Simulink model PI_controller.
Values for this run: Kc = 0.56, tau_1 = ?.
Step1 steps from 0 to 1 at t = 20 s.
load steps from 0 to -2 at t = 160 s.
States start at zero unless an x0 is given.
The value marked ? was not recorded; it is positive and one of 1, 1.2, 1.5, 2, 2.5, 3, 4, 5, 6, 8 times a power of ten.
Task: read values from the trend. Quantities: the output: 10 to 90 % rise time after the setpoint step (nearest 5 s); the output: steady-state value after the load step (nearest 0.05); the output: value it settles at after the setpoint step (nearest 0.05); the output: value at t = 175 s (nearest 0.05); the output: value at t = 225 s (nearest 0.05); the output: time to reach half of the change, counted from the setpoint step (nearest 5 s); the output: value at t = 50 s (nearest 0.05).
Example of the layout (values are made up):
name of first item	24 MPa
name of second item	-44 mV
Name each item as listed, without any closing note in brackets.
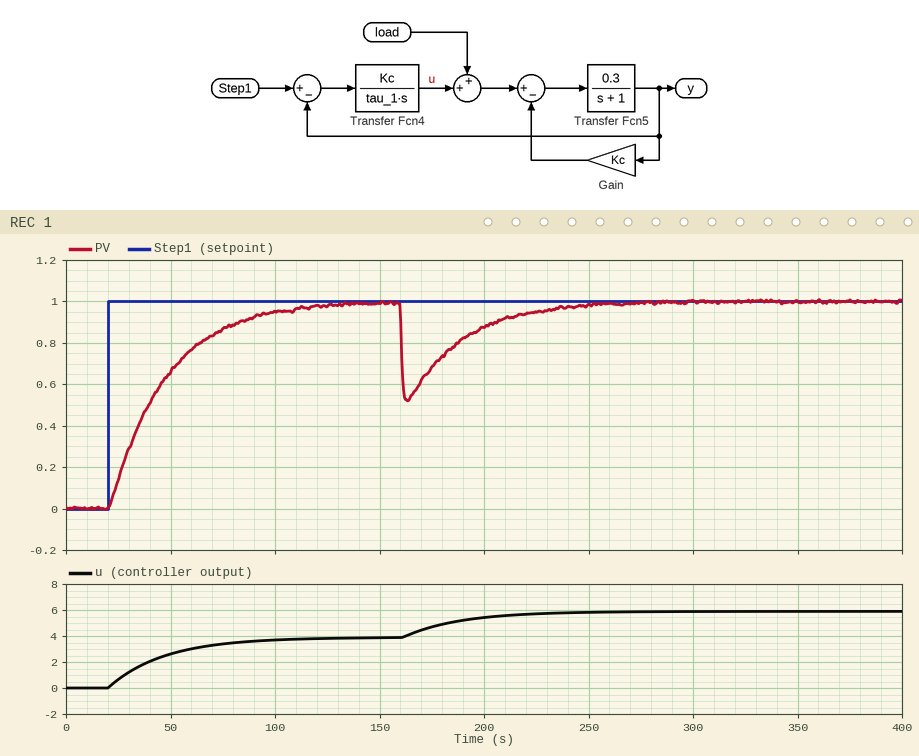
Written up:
the output: 10 to 90 % rise time after the setpoint step	60 s
the output: steady-state value after the load step	1.00
the output: value it settles at after the setpoint step	1.00
the output: value at t = 175 s	0.70
the output: value at t = 225 s	0.95
the output: time to reach half of the change, counted from the setpoint step	20 s
the output: value at t = 50 s	0.65
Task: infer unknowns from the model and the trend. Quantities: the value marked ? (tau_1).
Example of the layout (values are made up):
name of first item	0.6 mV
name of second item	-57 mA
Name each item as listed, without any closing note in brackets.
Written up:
the value marked ?	4
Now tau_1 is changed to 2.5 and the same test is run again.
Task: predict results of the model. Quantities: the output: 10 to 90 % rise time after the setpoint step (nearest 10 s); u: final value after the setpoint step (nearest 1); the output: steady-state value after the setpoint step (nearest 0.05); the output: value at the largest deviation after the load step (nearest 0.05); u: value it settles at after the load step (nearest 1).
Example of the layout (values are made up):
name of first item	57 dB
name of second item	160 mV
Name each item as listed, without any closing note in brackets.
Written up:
the output: 10 to 90 % rise time after the setpoint step	40 s
u: final value after the setpoint step	4
the output: steady-state value after the setpoint step	1.00
the output: value at the largest deviation after the load step	0.55
u: value it settles at after the load step	6
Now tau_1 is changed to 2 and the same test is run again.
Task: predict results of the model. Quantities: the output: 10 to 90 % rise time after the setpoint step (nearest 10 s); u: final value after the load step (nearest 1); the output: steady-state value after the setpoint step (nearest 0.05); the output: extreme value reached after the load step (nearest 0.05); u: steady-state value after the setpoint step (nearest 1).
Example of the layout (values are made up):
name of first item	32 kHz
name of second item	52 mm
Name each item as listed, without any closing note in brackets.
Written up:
the output: 10 to 90 % rise time after the setpoint step	30 s
u: final value after the load step	6
the output: steady-state value after the setpoint step	1.00
the output: extreme value reached after the load step	0.55
u: steady-state value after the setpoint step	4
